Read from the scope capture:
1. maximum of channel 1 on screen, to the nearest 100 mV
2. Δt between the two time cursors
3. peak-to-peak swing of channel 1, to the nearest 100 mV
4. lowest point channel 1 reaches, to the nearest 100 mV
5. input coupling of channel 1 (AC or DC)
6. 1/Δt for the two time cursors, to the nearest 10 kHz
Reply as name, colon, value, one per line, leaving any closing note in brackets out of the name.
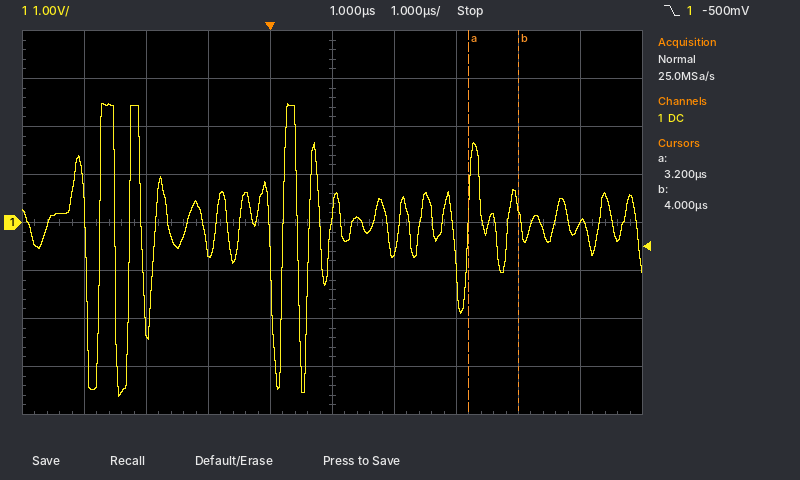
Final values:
maximum of channel 1 on screen, to the nearest 100 mV: 2.5 V
Δt between the two time cursors: 800 ns
peak-to-peak swing of channel 1, to the nearest 100 mV: 6.1 V
lowest point channel 1 reaches, to the nearest 100 mV: -3.6 V
input coupling of channel 1: DC
1/Δt for the two time cursors, to the nearest 10 kHz: 1.25 MHz
